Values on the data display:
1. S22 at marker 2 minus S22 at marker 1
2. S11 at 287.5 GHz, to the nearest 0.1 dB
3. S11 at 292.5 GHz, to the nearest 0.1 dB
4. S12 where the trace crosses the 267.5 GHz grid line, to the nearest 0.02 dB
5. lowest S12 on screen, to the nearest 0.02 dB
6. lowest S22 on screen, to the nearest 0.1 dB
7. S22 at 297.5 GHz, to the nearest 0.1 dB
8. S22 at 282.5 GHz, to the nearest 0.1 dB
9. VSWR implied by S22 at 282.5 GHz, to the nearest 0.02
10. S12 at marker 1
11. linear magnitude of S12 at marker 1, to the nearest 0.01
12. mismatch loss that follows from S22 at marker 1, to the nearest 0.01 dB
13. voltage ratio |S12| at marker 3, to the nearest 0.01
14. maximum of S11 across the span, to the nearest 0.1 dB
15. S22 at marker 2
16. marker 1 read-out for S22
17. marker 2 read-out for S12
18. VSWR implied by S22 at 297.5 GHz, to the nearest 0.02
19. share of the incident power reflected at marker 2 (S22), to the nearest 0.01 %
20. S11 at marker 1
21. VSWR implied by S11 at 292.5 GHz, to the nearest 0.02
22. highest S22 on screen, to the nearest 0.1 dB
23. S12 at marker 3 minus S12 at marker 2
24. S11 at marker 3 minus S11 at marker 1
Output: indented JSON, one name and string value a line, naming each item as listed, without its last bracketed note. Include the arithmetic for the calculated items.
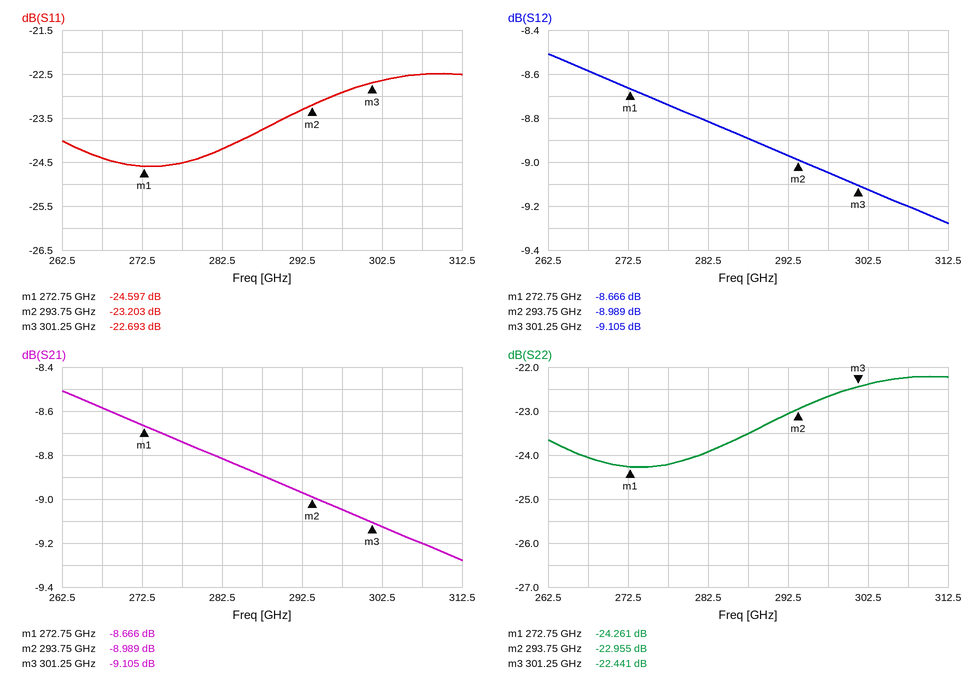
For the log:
{
  "S22 at marker 2 minus S22 at marker 1": "-22.955 − (-24.261) = 1.306 dB",
  "S11 at 287.5 GHz, to the nearest 0.1 dB": "-23.8 dB",
  "S11 at 292.5 GHz, to the nearest 0.1 dB": "-23.3 dB",
  "S12 where the trace crosses the 267.5 GHz grid line, to the nearest 0.02 dB": "-8.58 dB",
  "lowest S12 on screen, to the nearest 0.02 dB": "-9.28 dB",
  "lowest S22 on screen, to the nearest 0.1 dB": "-24.3 dB",
  "S22 at 297.5 GHz, to the nearest 0.1 dB": "-22.7 dB",
  "S22 at 282.5 GHz, to the nearest 0.1 dB": "-23.9 dB",
  "VSWR implied by S22 at 282.5 GHz, to the nearest 0.02": "|Γ| = 10^(-23.9/20) = 0.0638; VSWR = (1 + 0.0638)/(1 − 0.0638) ≈ 1.14",
  "S12 at marker 1": "-8.666 dB",
  "linear magnitude of S12 at marker 1, to the nearest 0.01": "10^(-8.666/20) ≈ 0.37",
  "mismatch loss that follows from S22 at marker 1, to the nearest 0.01 dB": "−10 log10(1 − 10^(-24.261/10)) ≈ 0.02 dB",
  "voltage ratio |S12| at marker 3, to the nearest 0.01": "10^(-9.105/20) ≈ 0.35",
  "maximum of S11 across the span, to the nearest 0.1 dB": "-22.5 dB",
  "S22 at marker 2": "-22.955 dB",
  "marker 1 read-out for S22": "-24.261 dB",
  "marker 2 read-out for S12": "-8.989 dB",
  "VSWR implied by S22 at 297.5 GHz, to the nearest 0.02": "|Γ| = 10^(-22.7/20) = 0.0733; VSWR = (1 + 0.0733)/(1 − 0.0733) ≈ 1.16",
  "share of the incident power reflected at marker 2 (S22), to the nearest 0.01 %": "10^(-22.955/10) ≈ 0.51 %",
  "S11 at marker 1": "-24.597 dB",
  "VSWR implied by S11 at 292.5 GHz, to the nearest 0.02": "|Γ| = 10^(-23.3/20) = 0.0684; VSWR = (1 + 0.0684)/(1 − 0.0684) ≈ 1.15, so 1.14 to the nearest 0.02",
  "highest S22 on screen, to the nearest 0.1 dB": "-22.2 dB",
  "S12 at marker 3 minus S12 at marker 2": "-9.105 − (-8.989) = -0.116 dB",
  "S11 at marker 3 minus S11 at marker 1": "-22.693 − (-24.597) = 1.904 dB"
}
